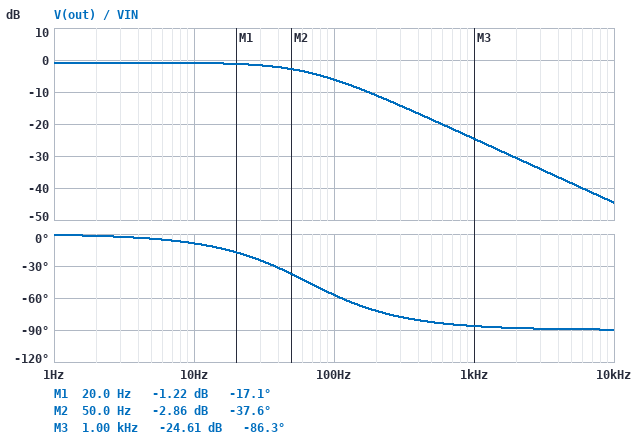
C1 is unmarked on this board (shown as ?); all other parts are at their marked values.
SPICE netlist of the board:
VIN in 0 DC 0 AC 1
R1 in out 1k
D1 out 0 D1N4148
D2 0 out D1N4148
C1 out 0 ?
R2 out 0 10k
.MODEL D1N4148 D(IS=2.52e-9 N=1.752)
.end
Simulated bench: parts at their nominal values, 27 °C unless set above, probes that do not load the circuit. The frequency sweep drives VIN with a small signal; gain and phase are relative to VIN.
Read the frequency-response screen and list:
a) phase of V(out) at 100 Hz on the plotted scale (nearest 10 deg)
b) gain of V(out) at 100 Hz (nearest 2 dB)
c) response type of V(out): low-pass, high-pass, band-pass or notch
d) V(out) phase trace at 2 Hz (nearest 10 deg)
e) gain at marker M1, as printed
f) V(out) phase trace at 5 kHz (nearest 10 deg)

-60 deg
-6 dB
low-pass
0 deg
-1.22 dB
-90 deg
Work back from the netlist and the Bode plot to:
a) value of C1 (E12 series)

2.7 µF
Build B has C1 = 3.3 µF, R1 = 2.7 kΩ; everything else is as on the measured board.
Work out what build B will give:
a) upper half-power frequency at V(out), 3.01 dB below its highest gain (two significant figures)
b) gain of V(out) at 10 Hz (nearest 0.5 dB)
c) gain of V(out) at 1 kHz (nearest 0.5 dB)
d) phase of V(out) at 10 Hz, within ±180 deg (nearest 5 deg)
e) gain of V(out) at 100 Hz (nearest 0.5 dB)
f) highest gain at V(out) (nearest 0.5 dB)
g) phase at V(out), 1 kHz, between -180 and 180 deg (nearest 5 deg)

23 Hz
-3.0 dB
-35.0 dB
-25 deg
-15.0 dB
-2.0 dB
-90 deg
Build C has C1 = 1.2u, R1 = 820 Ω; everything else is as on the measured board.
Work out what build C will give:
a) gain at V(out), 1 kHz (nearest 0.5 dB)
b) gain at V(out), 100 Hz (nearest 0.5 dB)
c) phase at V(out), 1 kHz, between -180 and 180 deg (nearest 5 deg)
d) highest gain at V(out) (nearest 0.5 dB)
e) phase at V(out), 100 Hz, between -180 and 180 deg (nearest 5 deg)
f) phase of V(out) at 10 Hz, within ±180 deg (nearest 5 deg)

-16.0 dB
-2.0 dB
-80 deg
-0.5 dB
-30 deg
-5 deg
